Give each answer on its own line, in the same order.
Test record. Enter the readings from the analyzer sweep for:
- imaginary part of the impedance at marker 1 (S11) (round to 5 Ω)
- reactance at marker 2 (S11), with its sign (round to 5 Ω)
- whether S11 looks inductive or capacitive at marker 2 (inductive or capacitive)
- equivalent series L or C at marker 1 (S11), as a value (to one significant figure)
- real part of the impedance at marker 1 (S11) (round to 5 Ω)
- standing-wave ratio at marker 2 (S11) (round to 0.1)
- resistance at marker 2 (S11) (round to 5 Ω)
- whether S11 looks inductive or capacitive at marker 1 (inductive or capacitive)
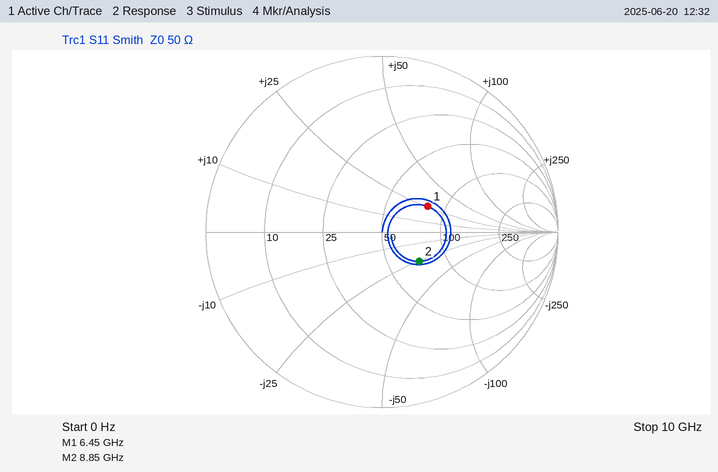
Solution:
+25 Ω
-25 Ω
capacitive
600 pH
80 Ω
1.7
70 Ω
inductive
